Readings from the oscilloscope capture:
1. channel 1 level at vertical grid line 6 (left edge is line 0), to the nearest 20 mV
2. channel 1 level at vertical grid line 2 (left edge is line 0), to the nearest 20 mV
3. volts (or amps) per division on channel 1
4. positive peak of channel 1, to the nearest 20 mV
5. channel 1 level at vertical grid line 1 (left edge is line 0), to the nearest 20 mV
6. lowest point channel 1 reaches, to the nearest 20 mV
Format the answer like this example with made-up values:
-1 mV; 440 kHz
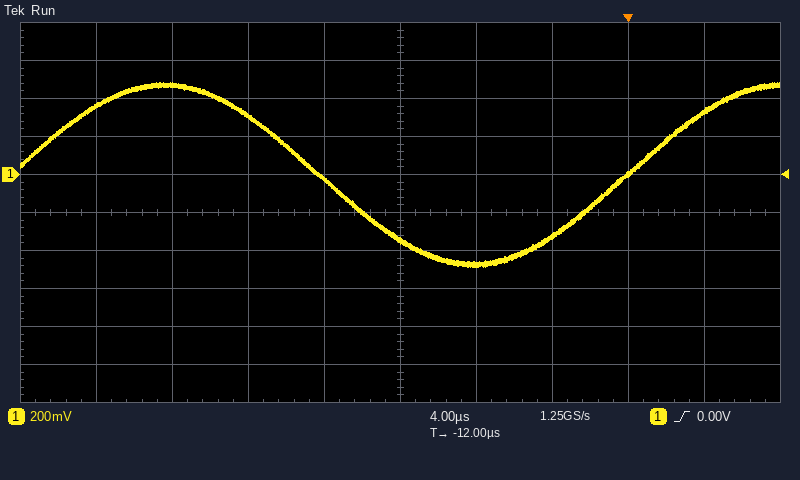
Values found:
-480 mV; 480 mV; 200 mV; 480 mV; 360 mV; -480 mV
